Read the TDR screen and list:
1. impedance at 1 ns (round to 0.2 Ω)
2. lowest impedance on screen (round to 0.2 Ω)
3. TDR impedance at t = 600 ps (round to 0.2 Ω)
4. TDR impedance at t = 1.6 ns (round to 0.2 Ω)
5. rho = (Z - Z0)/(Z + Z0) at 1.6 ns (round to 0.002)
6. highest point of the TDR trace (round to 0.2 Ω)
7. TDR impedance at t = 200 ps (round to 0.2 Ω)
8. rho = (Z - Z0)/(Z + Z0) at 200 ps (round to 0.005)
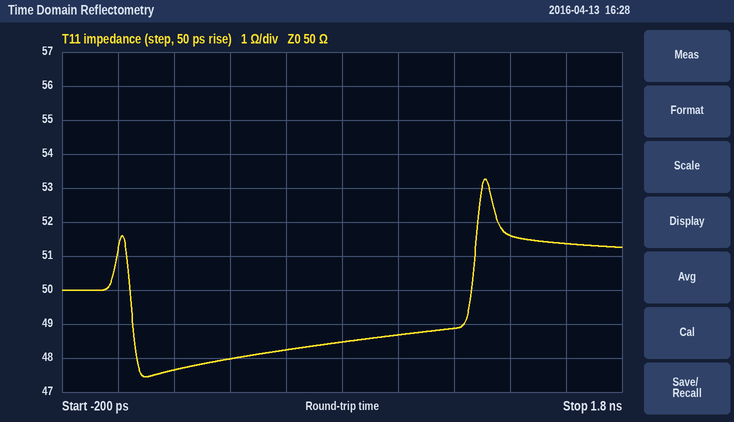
48.6 Ω
47.4 Ω
48.2 Ω
51.4 Ω
+0.014
53.2 Ω
47.6 Ω
-0.025
